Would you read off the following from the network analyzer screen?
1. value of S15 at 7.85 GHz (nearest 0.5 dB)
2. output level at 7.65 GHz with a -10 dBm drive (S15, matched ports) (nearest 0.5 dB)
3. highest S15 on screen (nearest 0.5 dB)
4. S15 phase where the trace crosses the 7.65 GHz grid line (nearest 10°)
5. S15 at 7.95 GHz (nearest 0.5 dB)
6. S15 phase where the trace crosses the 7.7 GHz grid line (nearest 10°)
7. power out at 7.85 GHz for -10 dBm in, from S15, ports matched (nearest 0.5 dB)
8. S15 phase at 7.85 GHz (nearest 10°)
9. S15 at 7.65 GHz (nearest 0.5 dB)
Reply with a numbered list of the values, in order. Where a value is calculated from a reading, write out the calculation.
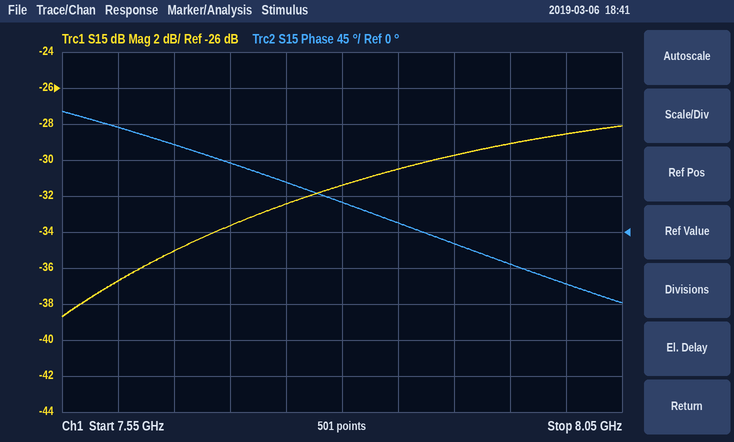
1. -30.5 dB
2. -10 dBm + (-35.0 dB) = -45.0 dBm
3. -28.0 dB
4. 110°
5. -29.0 dB
6. 90°
7. -10 dBm + (-30.5 dB) = -40.5 dBm
8. 10°
9. -35.0 dB
